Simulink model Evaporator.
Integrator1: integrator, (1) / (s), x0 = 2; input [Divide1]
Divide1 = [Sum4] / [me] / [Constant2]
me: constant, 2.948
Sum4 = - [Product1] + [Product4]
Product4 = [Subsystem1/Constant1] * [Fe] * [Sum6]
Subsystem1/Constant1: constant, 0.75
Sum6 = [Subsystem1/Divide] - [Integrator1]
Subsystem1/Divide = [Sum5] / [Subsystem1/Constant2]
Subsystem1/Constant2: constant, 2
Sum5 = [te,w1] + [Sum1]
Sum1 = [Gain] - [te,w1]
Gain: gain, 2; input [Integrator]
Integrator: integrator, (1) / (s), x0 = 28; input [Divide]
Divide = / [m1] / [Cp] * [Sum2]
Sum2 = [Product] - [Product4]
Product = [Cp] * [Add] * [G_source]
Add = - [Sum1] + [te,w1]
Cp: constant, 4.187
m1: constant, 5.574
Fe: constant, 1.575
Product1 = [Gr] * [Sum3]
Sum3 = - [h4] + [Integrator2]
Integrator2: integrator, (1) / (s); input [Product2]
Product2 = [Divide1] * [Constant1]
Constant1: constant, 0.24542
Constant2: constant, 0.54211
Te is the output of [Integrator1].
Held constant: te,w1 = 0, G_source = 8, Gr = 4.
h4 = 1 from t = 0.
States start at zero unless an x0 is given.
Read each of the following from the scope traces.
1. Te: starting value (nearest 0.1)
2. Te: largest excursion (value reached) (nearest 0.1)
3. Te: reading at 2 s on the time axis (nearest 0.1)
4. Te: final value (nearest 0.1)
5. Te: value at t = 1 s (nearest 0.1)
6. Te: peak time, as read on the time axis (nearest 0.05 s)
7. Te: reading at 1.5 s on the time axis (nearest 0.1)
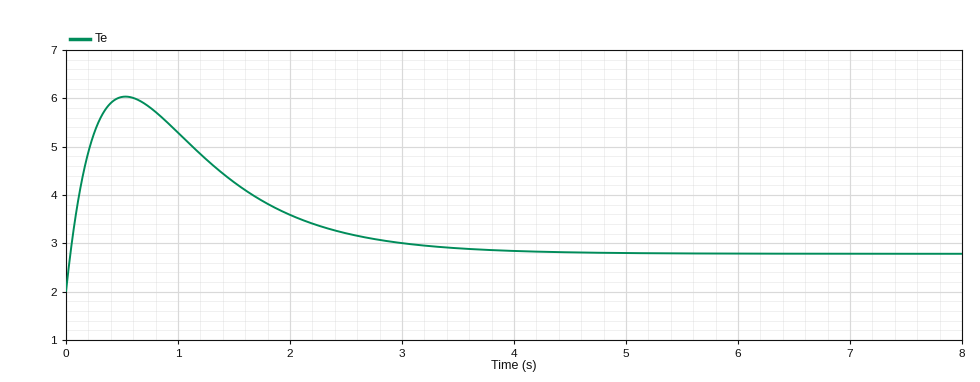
2.0
6.0
3.6
2.8
5.3
0.55 s
4.3
